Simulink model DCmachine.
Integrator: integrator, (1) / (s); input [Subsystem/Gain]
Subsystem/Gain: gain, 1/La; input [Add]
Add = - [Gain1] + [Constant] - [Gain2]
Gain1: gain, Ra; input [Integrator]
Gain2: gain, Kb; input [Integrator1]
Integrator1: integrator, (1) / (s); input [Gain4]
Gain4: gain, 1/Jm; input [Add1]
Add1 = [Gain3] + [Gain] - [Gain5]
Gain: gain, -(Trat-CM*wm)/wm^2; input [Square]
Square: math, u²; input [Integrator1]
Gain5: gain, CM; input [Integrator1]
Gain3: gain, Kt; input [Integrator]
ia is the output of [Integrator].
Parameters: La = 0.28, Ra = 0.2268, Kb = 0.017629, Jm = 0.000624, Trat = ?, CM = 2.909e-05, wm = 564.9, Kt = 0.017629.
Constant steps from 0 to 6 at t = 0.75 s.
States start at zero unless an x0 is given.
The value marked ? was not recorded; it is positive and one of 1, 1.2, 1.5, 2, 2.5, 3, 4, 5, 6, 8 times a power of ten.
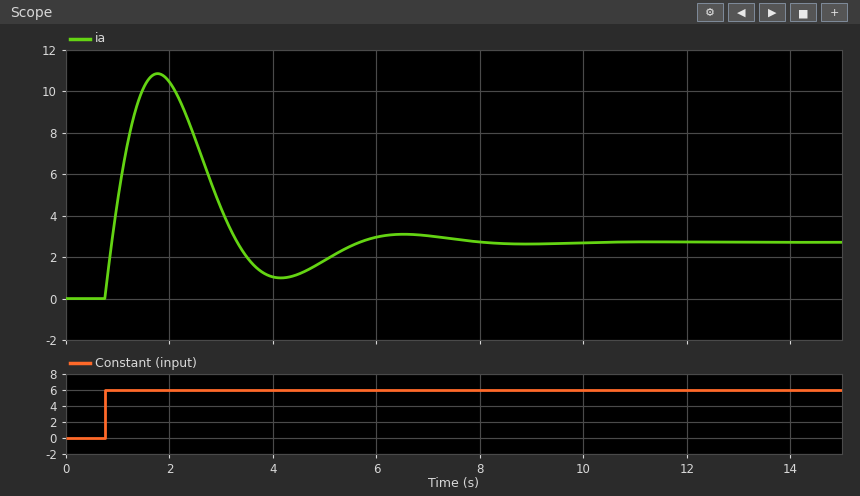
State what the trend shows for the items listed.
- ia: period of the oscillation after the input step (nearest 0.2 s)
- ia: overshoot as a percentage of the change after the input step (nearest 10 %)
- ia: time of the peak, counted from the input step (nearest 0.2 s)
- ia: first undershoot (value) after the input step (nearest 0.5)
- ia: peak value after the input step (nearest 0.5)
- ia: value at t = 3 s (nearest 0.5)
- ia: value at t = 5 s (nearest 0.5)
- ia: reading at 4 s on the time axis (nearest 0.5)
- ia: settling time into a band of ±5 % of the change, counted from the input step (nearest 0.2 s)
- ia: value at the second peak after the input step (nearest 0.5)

4.8 s
300 %
1.0 s
1.0
11.0
4.5
2.0
1.0
6.8 s
3.0
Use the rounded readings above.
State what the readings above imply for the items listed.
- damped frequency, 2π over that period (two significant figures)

1.3 rad/s
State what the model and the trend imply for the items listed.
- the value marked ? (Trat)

0.15
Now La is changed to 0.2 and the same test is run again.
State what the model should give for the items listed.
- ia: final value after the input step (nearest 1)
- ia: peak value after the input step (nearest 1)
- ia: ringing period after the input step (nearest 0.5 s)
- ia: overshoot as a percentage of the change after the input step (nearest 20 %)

3
12
4.0 s
340 %
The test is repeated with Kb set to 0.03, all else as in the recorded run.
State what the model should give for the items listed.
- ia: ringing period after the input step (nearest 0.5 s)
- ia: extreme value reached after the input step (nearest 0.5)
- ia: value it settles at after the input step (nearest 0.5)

3.5 s
9.0
1.0
